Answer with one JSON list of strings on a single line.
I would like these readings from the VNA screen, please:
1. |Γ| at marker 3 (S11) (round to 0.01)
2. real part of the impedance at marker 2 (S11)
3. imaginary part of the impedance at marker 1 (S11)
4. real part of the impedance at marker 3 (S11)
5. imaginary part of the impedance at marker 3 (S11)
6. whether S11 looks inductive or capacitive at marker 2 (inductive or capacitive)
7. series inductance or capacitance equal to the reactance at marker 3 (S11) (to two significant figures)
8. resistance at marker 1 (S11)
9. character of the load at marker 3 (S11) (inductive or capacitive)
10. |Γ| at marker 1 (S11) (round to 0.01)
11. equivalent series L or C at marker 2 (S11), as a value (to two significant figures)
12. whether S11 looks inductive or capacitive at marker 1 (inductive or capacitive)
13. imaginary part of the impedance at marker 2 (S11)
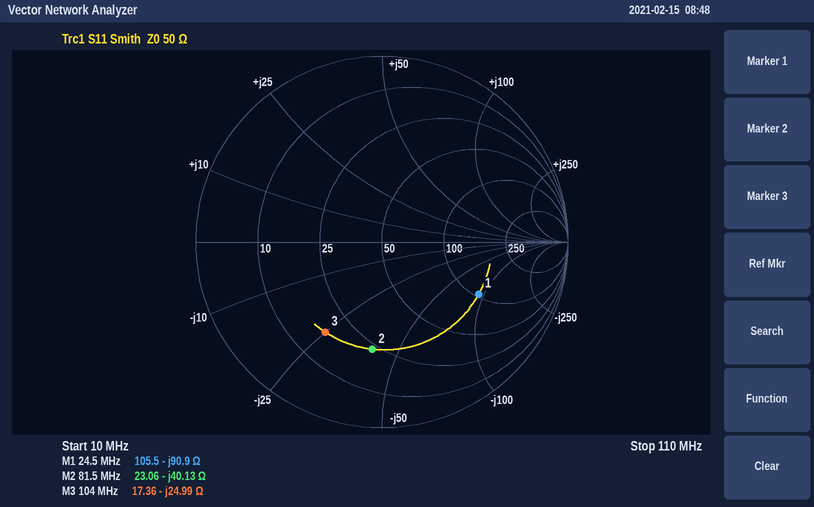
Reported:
["0.57", "23.06 Ω", "-90.9 Ω", "17.36 Ω", "-24.99 Ω", "capacitive", "61 pF", "105.5 Ω", "capacitive", "0.59", "49 pF", "capacitive", "-40.13 Ω"]
